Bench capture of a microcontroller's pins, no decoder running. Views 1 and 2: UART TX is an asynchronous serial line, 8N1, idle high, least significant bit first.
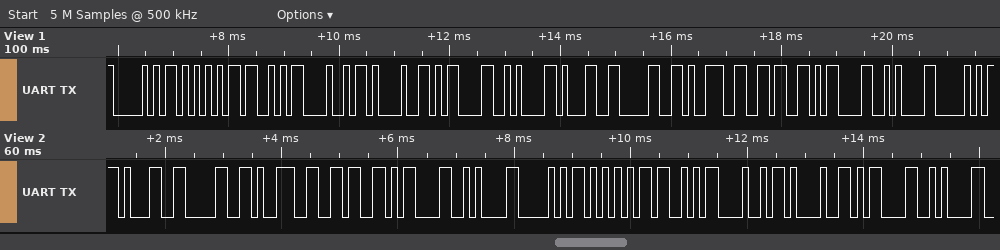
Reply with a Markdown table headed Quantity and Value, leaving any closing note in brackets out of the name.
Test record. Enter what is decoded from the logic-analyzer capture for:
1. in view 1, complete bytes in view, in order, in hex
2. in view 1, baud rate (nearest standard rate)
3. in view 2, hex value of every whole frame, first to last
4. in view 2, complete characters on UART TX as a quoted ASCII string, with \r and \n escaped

| Quantity | Value |
|---|---|
| in view 1, complete bytes in view, in order, in hex | 50 55 53 48 21 0D 0A 31 30 39 36 0D 0A 50 |
| in view 1, baud rate | 9600 baud |
| in view 2, hex value of every whole frame, first to last | 31 30 39 36 0D 0A 50 55 53 48 21 0D 0A |
| in view 2, complete characters on UART TX as a quoted ASCII string, with \r and \n escaped | "1096\r\nPUSH!\r\n" |
